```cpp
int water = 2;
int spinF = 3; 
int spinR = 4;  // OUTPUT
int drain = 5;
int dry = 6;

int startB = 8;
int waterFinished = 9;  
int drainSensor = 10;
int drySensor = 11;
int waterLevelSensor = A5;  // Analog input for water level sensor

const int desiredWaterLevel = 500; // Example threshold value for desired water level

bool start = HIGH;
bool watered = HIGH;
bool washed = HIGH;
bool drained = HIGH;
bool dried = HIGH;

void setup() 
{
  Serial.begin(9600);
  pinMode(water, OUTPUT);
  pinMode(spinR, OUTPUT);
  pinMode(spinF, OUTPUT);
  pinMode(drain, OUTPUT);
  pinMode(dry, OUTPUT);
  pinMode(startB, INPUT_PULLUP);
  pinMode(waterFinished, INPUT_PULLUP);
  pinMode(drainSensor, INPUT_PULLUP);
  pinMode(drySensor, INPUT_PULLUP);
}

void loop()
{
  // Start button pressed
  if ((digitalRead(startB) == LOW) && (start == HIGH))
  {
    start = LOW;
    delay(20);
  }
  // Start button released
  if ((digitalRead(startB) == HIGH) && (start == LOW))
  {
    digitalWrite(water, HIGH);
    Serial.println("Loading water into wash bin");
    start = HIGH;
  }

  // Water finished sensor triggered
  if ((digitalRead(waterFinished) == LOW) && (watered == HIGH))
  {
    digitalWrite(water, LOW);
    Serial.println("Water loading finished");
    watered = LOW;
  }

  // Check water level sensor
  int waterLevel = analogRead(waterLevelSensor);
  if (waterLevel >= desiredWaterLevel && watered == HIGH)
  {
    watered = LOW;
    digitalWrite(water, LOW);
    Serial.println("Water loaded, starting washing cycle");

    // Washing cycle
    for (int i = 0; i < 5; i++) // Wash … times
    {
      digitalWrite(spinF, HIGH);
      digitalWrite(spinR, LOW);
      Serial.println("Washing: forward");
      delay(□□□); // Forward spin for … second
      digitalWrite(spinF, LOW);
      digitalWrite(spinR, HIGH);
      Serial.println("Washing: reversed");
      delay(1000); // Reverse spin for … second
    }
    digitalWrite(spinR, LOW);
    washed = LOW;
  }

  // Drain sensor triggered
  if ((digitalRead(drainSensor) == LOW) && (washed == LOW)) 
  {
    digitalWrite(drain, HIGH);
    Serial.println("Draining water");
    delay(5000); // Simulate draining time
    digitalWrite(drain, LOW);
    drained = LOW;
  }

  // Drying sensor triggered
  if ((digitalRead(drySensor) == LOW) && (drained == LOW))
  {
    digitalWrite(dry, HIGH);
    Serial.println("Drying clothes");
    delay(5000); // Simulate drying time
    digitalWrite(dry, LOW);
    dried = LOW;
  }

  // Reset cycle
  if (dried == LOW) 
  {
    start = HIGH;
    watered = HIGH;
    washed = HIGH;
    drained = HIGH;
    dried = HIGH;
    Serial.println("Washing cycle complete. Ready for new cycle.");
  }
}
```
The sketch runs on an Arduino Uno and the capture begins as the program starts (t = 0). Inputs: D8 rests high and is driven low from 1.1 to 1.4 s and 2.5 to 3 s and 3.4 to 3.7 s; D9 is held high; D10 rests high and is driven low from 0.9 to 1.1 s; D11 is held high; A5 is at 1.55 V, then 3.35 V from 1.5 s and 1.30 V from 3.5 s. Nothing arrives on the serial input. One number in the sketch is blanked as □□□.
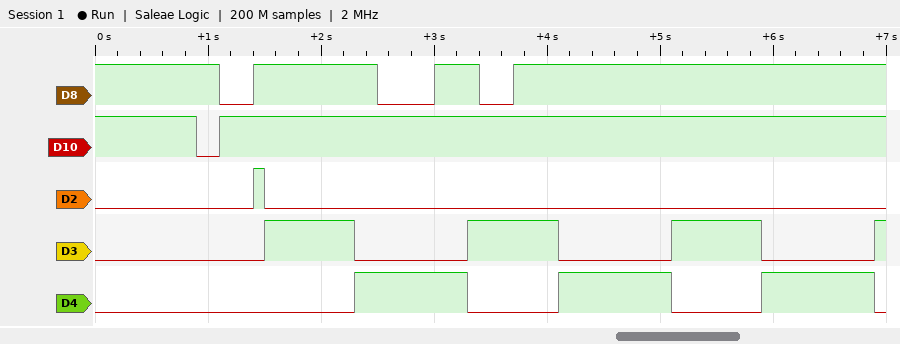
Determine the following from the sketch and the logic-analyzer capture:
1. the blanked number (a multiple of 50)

800
